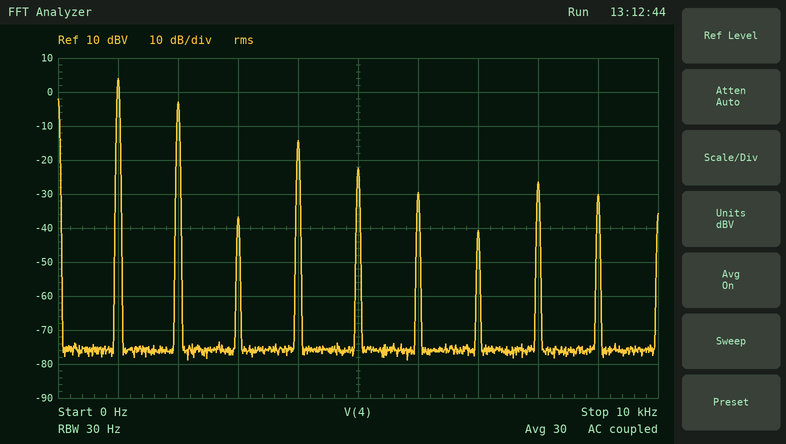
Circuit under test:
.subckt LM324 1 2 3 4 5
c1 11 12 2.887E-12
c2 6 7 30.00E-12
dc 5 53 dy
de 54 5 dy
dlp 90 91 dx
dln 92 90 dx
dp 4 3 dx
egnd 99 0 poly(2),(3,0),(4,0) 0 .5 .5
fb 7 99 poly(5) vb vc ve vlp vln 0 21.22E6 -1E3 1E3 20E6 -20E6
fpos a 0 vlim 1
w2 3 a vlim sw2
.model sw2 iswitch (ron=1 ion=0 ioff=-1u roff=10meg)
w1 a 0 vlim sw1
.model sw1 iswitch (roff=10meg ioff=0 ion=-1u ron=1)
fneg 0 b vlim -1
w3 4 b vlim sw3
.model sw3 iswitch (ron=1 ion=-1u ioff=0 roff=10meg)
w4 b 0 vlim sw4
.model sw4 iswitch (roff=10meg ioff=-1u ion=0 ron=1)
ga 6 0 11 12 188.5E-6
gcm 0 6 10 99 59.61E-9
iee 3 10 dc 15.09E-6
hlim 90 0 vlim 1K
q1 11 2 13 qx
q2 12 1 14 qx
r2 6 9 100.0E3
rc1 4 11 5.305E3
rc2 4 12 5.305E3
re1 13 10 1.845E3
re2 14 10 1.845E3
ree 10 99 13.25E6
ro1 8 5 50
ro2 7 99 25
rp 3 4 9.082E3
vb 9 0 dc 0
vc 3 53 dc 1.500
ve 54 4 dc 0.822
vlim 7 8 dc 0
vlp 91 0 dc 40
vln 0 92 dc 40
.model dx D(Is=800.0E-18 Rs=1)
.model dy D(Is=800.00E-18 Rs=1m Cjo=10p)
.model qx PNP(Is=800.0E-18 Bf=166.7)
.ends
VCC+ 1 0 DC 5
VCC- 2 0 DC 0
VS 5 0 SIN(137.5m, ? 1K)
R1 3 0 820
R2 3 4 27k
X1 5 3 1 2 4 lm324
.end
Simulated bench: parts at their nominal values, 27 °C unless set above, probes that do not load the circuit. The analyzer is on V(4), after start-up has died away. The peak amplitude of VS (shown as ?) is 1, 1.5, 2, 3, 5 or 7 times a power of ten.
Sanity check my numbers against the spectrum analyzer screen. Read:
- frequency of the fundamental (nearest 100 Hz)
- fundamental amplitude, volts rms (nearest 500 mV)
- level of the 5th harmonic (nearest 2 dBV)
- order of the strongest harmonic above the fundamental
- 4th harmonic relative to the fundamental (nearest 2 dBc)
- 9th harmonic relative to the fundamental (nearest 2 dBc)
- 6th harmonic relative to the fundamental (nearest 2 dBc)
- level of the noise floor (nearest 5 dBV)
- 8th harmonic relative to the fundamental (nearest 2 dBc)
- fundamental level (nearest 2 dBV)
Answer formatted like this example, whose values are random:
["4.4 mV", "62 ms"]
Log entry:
["1.0 kHz", "1.5 V", "-22 dBV", "2", "-18 dBc", "-34 dBc", "-34 dBc", "-75 dBV", "-30 dBc", "4 dBV"]
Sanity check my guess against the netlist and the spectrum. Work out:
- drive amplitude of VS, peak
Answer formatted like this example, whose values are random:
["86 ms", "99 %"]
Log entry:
["150 mV"]
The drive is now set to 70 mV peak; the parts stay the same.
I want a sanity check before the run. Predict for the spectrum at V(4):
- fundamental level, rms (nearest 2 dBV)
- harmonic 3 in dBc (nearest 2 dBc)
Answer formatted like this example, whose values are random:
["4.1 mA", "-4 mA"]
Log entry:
["-4 dBV", "-22 dBc"]
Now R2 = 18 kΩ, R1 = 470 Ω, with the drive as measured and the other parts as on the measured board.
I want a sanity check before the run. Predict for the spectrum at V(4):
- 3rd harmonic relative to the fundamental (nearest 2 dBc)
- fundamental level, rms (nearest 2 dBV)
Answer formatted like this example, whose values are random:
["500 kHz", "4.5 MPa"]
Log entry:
["-22 dBc", "4 dBV"]
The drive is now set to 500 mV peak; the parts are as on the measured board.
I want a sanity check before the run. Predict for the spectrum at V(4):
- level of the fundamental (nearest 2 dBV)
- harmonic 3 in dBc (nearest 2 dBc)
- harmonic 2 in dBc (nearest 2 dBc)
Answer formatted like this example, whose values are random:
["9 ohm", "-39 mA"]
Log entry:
["6 dBV", "-10 dBc", "-16 dBc"]
